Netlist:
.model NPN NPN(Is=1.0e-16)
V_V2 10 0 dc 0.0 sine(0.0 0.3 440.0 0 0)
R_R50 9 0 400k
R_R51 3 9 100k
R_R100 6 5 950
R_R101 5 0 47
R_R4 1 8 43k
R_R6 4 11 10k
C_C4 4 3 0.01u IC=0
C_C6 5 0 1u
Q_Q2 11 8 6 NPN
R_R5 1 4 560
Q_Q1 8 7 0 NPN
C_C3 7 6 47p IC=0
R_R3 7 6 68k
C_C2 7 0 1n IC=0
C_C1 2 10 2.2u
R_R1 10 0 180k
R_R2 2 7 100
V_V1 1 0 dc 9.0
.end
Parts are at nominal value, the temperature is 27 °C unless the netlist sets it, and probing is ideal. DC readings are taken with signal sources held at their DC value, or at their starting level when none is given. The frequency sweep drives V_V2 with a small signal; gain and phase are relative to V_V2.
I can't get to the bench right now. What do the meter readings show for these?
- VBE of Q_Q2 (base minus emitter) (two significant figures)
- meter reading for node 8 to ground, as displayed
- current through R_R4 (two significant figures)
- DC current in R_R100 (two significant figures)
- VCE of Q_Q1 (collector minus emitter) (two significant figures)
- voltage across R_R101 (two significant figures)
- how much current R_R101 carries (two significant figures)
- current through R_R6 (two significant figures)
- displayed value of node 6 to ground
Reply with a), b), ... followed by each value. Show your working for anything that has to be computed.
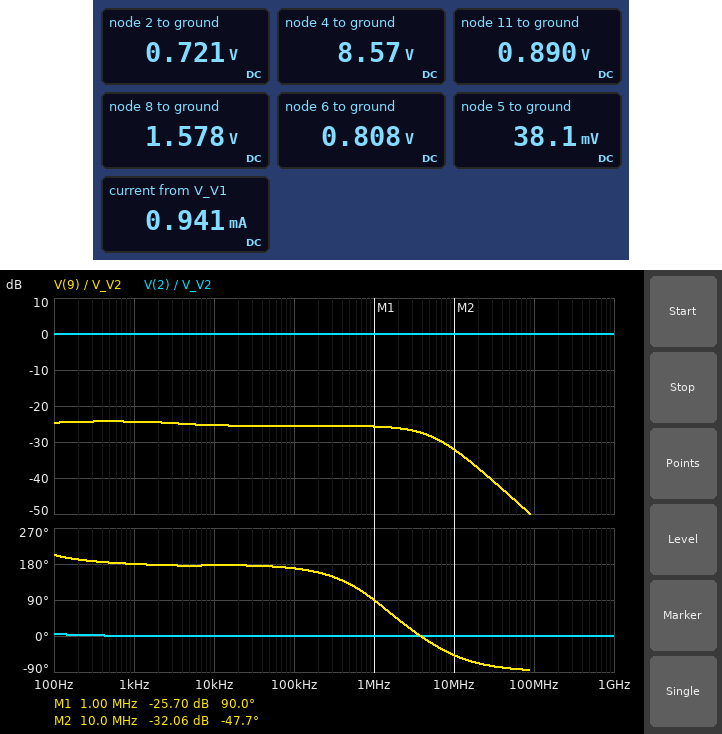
a) 1.578 V - 808 mV = 770 mV
b) 1.578 V
c) (9 V - 1.578 V) / 43 kΩ = 170 µA
d) (808 mV - 38.1 mV) / 950 Ω = 810 µA
e) 1.578 V = 1.6 V
f) 38.1 mV = 38 mV
g) (38.1 mV) / 47 Ω = 810 µA
h) (8.57 V - 890 mV) / 10 kΩ = 770 µA
i) 0.808 V
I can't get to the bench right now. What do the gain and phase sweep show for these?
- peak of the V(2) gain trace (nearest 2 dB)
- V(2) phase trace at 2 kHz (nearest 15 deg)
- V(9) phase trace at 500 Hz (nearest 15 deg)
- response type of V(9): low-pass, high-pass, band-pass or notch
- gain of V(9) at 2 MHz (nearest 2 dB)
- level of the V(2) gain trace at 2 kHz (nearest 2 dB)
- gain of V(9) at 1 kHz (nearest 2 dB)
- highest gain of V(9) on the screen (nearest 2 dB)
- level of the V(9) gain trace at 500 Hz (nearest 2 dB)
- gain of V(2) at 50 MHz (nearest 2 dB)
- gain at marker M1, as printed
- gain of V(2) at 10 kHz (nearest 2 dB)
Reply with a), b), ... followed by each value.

a) 0 dB
b) 0 deg
c) 180 deg
d) low-pass
e) -26 dB
f) 0 dB
g) -24 dB
h) -24 dB
i) -24 dB
j) 0 dB
k) -25.70 dB
l) 0 dB
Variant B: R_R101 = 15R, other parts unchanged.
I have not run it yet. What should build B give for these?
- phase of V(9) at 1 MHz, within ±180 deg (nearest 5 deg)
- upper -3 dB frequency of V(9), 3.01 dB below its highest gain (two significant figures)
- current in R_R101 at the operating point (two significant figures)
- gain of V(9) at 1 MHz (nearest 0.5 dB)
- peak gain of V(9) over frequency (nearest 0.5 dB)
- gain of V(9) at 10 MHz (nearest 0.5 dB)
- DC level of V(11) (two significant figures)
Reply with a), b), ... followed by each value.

a) 110 deg
b) 1.4 MHz
c) 830 µA
d) -24.0 dB
e) -22.0 dB
f) -34.5 dB
g) 870 mV
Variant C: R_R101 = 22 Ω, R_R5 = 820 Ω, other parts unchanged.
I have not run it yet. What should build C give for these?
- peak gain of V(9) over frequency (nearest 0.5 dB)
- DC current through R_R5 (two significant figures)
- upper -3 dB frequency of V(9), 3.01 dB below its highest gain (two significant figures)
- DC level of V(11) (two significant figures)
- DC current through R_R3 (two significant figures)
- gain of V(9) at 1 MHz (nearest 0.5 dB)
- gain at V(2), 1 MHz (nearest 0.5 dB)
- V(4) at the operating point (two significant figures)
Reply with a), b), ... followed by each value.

a) -18.0 dB
b) 750 µA
c) 1.3 MHz
d) 860 mV
e) 1.1 µA
f) -20.5 dB
g) 0 dB
h) 8.4 V
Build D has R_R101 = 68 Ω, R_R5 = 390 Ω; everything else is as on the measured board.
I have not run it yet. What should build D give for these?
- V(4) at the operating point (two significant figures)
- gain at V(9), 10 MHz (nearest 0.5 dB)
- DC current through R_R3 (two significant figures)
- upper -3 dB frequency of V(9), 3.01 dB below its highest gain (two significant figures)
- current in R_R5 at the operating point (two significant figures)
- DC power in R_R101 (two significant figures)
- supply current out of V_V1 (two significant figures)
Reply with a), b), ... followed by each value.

a) 8.7 V
b) -30.5 dB
c) 1.4 µA
d) 7.4 MHz
e) 780 µA
f) 44 µW
g) 950 µA
